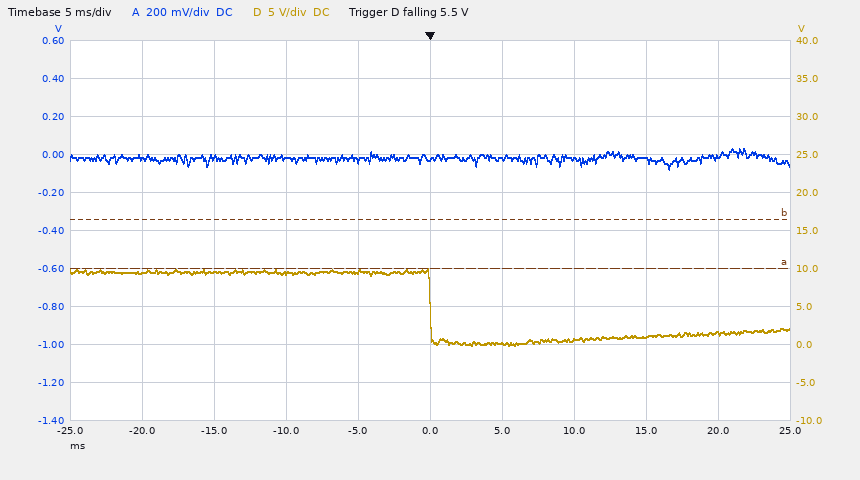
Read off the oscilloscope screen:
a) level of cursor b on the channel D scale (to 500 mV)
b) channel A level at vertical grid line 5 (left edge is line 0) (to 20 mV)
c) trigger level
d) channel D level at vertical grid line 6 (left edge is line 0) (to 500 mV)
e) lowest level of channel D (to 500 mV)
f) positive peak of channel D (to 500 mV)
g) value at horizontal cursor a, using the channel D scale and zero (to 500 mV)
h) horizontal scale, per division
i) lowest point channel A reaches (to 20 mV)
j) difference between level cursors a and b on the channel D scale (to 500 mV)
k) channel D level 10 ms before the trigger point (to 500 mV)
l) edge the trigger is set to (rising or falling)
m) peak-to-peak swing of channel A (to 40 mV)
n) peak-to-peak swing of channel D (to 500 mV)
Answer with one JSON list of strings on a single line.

["16.5 V", "-20 mV", "5.5 V", "0.0 V", "0.0 V", "10.0 V", "10.0 V", "5 ms", "-80 mV", "6.5 V", "9.5 V", "falling", "120 mV", "10.0 V"]
